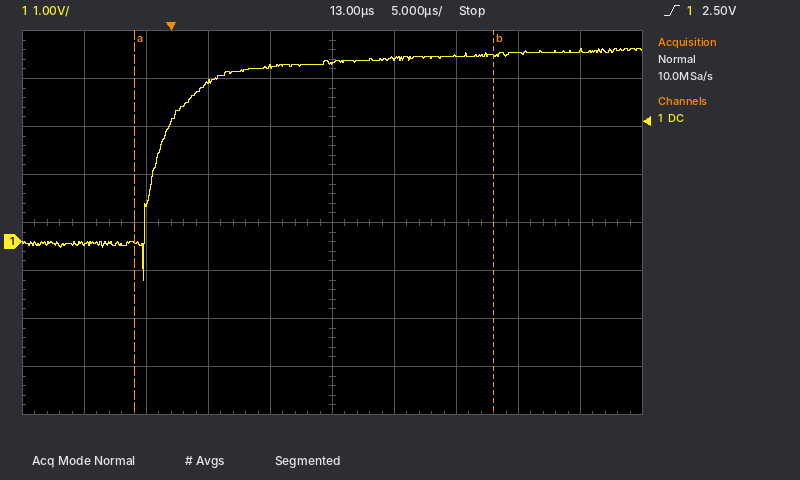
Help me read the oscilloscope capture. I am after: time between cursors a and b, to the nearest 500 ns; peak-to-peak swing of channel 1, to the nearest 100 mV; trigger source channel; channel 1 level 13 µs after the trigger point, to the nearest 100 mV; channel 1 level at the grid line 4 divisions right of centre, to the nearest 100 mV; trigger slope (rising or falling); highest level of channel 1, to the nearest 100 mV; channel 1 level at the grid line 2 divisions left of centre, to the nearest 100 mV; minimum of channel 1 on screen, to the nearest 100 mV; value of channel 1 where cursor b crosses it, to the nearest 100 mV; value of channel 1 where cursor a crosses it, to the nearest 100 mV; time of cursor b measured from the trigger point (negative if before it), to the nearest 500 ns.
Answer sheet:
29.0 µs
4.8 V
channel 1
3.7 V
4.0 V
rising
4.0 V
3.3 V
-800 mV
3.9 V
0.0 V
+26.0 µs
